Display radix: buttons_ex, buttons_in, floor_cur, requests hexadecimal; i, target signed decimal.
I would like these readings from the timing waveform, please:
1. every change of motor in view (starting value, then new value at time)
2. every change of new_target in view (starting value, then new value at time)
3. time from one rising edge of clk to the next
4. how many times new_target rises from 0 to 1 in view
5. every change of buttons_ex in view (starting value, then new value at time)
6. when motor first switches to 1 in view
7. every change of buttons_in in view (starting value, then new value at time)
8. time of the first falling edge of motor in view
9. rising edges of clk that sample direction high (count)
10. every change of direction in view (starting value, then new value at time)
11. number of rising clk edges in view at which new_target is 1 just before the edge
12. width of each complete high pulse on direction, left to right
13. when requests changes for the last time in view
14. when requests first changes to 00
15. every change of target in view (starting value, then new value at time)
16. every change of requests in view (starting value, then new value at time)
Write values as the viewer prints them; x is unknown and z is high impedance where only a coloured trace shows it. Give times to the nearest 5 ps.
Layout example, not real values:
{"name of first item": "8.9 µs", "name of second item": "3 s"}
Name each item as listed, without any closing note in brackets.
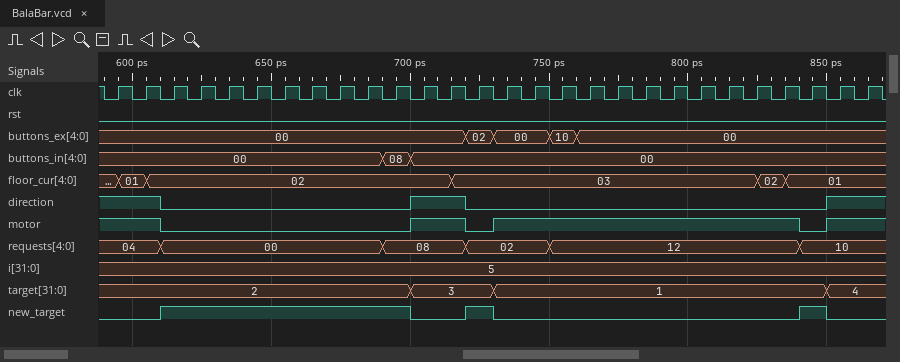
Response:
{"every change of motor in view": "1, 0 at 610 ps, 1 at 700 ps, 0 at 720 ps, 1 at 730 ps, 0 at 840 ps, 1 at 850 ps", "every change of new_target in view": "0, 1 at 610 ps, 0 at 700 ps, 1 at 720 ps, 0 at 730 ps, 1 at 840 ps, 0 at 850 ps", "time from one rising edge of clk to the next": "10 ps", "how many times new_target rises from 0 to 1 in view": "3", "every change of buttons_ex in view": "00, 02 at 720 ps, 00 at 730 ps, 10 at 750 ps, 00 at 760 ps", "when motor first switches to 1 in view": "700 ps", "every change of buttons_in in view": "00, 08 at 690 ps, 00 at 700 ps", "time of the first falling edge of motor in view": "610 ps", "rising edges of clk that sample direction high": "6", "every change of direction in view": "1, 0 at 610 ps, 1 at 700 ps, 0 at 720 ps, 1 at 850 ps", "number of rising clk edges in view at which new_target is 1 just before the edge": "11", "width of each complete high pulse on direction, left to right": "20 ps", "when requests changes for the last time in view": "840 ps", "when requests first changes to 00": "610 ps", "every change of target in view": "2, 3 at 700 ps, 1 at 730 ps, 4 at 850 ps", "every change of requests in view": "04, 00 at 610 ps, 08 at 690 ps, 02 at 720 ps, 12 at 750 ps, 10 at 840 ps"}
